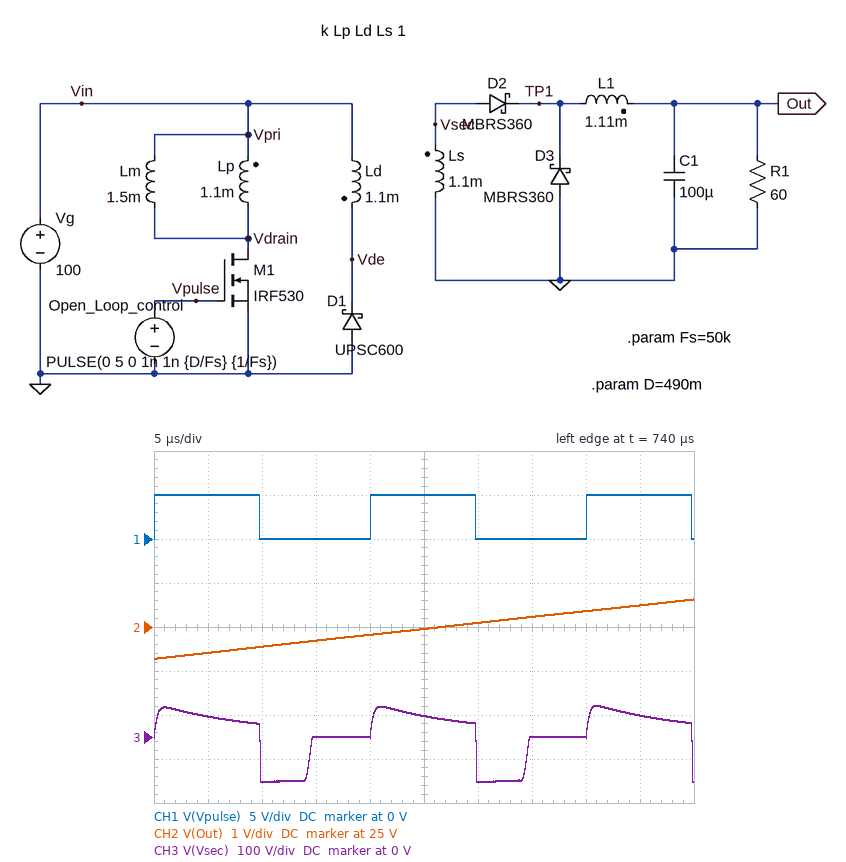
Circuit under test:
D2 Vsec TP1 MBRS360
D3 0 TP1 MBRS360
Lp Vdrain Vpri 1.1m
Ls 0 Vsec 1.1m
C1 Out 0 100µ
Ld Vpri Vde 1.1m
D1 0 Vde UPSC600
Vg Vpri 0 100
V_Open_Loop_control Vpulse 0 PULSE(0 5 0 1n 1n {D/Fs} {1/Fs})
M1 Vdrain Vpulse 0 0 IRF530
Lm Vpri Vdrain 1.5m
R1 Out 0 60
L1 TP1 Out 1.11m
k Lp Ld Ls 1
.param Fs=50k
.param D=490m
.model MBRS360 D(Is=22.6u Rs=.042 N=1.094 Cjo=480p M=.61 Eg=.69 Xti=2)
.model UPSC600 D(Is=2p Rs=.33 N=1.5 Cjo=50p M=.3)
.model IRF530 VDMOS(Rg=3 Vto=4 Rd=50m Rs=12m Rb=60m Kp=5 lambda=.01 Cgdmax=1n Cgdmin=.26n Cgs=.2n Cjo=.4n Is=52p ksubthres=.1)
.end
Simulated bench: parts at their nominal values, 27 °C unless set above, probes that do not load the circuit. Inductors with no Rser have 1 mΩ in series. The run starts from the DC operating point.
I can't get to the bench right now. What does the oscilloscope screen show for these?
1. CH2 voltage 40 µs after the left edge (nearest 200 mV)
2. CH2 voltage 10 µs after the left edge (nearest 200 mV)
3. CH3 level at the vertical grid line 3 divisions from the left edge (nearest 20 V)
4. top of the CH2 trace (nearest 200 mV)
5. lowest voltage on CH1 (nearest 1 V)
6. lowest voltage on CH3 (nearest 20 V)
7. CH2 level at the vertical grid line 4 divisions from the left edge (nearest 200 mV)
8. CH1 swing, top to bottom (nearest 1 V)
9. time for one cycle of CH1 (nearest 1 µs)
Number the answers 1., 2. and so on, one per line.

1. 25.4 V
2. 24.6 V
3. 0 V
4. 25.6 V
5. 0 V
6. -100 V
7. 24.8 V
8. 5 V
9. 20 µs
